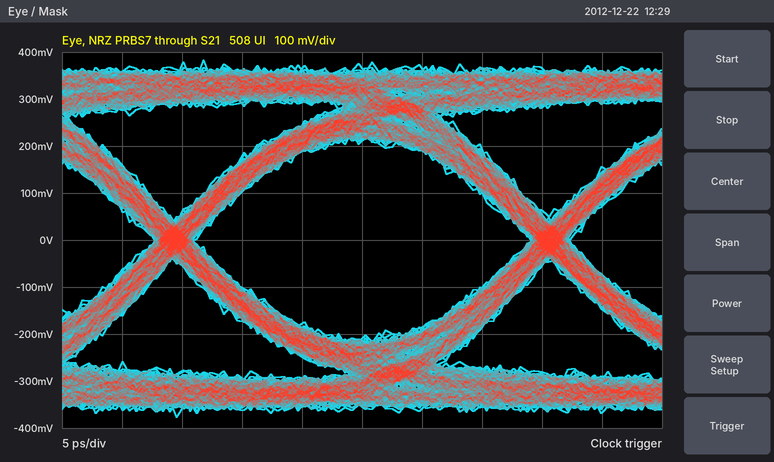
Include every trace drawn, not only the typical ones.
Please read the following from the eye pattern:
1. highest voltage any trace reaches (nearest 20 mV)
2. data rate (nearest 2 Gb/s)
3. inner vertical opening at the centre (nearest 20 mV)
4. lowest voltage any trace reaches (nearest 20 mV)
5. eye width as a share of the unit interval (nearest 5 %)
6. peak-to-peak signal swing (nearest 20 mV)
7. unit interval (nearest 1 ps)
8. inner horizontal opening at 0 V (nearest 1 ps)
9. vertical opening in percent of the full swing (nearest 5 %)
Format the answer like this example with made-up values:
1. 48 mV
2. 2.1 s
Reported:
1. 380 mV
2. 32 Gb/s
3. 420 mV
4. -380 mV
5. 90 %
6. 760 mV
7. 31 ps
8. 28 ps
9. 55 %
